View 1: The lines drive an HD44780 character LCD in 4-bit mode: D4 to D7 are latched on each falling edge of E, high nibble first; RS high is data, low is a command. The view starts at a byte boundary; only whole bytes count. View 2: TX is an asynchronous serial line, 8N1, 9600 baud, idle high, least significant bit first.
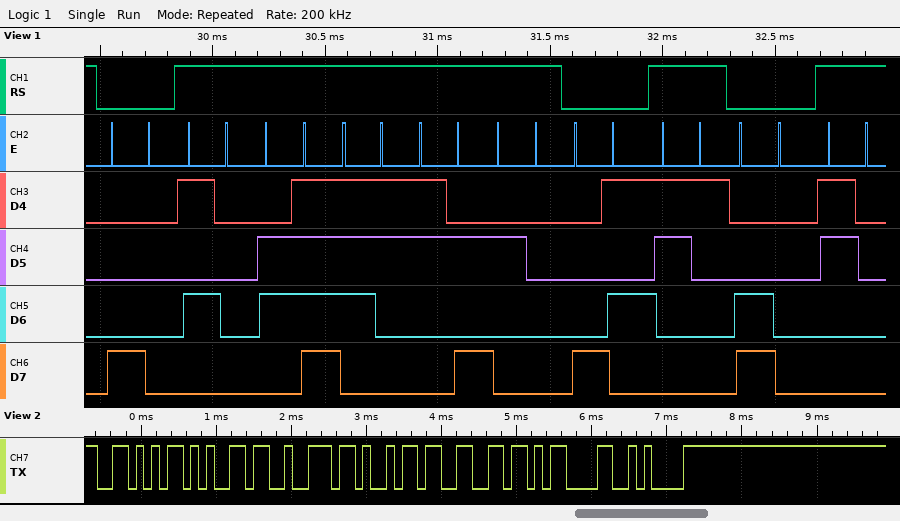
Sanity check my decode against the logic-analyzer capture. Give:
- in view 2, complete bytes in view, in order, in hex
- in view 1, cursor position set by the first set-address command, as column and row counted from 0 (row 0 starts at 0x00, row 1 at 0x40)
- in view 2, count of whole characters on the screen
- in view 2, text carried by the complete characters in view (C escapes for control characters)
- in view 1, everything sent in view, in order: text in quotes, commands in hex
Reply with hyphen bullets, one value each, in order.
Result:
- 56 65 72 69 66 0D 0A
- column 0, row 0
- 7
- "Verif\r\n"
- 0x80 "Pos: " 0x85 "1" 0xC0 "0"
